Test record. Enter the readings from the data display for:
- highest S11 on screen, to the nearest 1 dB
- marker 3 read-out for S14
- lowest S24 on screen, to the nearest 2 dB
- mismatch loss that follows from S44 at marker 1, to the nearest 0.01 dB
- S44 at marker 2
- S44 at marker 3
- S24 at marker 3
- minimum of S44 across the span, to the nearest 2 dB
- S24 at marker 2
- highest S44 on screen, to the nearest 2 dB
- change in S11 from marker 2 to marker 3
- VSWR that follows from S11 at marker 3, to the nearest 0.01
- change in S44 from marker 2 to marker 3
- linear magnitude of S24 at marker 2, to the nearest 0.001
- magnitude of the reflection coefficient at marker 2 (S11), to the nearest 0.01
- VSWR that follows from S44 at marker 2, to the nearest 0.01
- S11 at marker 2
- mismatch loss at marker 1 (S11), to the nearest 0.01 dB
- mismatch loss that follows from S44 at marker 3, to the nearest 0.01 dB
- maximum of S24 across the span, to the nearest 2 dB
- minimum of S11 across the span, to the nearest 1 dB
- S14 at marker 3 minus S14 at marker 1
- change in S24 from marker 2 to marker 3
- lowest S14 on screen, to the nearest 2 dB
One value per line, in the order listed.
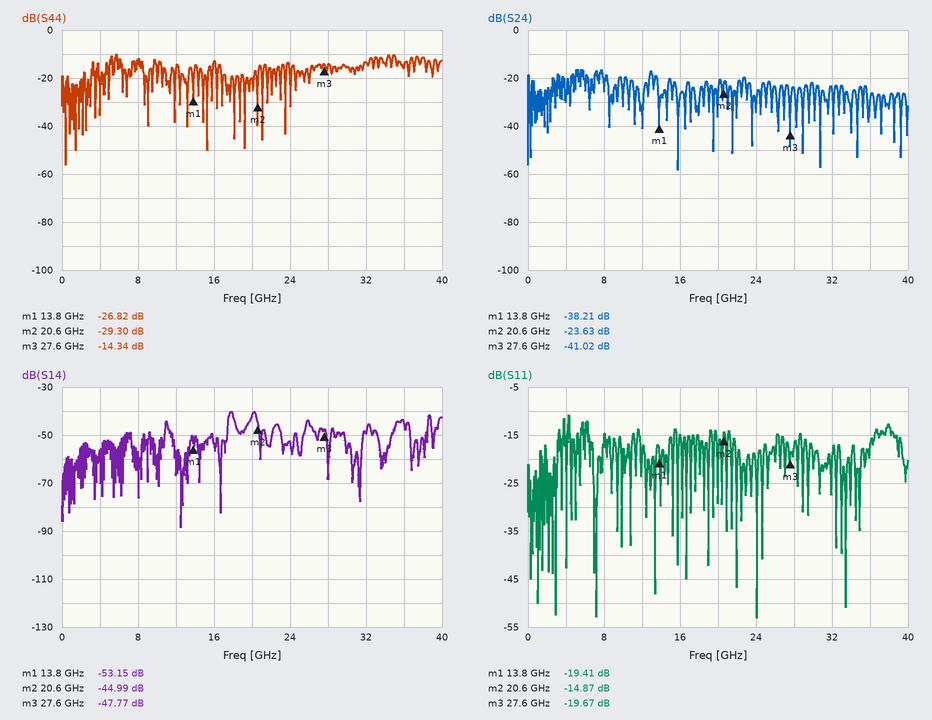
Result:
-11 dB
-47.77 dB
-58 dB
0.01 dB
-29.30 dB
-14.34 dB
-41.02 dB
-56 dB
-23.63 dB
-10 dB
-4.80 dB
1.23
14.96 dB
0.066
0.18
1.07
-14.87 dB
0.05 dB
0.16 dB
-16 dB
-53 dB
5.38 dB
-17.39 dB
-88 dB
